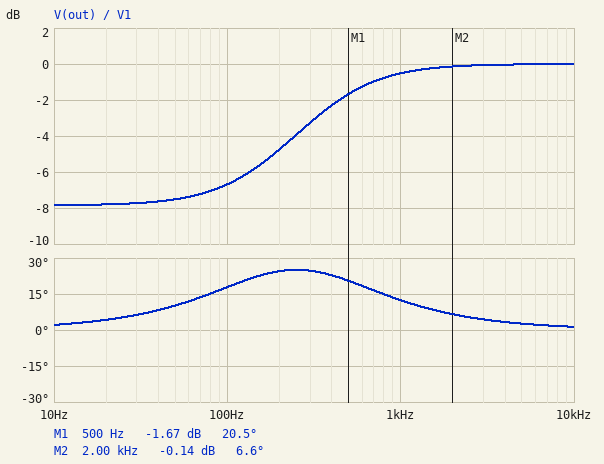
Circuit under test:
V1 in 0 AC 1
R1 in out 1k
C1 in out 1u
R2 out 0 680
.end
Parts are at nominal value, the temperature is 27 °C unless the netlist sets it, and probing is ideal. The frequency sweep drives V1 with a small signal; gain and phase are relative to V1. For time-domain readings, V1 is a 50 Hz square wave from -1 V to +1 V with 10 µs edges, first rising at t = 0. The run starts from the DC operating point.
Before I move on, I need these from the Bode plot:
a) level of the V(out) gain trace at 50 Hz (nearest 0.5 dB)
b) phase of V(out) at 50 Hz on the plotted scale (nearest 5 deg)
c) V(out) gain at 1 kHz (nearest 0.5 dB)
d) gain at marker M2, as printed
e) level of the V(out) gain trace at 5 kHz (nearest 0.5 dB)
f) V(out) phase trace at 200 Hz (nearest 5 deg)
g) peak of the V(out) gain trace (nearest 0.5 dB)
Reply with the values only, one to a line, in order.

-7.5 dB
10 deg
-0.5 dB
-0.14 dB
0 dB
25 deg
0 dB
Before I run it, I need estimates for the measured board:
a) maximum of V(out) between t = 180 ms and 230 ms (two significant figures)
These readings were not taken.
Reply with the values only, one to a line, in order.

1.6 V
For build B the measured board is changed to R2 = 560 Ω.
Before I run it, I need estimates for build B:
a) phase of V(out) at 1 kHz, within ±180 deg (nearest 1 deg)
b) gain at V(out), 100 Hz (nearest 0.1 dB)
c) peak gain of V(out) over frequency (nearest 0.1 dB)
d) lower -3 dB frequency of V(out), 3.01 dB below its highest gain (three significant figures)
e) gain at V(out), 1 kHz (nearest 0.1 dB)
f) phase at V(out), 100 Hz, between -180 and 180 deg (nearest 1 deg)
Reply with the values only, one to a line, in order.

15 deg
-7.7 dB
0 dB
382 Hz
-0.7 dB
19 deg
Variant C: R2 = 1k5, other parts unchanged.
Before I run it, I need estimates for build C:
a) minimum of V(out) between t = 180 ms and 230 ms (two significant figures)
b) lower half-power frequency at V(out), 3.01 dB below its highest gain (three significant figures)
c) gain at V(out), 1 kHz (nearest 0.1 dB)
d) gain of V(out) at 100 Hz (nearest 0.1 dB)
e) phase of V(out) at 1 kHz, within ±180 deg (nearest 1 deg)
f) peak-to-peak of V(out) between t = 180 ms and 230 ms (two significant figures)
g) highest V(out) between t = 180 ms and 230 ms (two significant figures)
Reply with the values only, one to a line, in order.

-1.4 V
140 Hz
-0.2 dB
-3.6 dB
6 deg
2.8 V
1.4 V
